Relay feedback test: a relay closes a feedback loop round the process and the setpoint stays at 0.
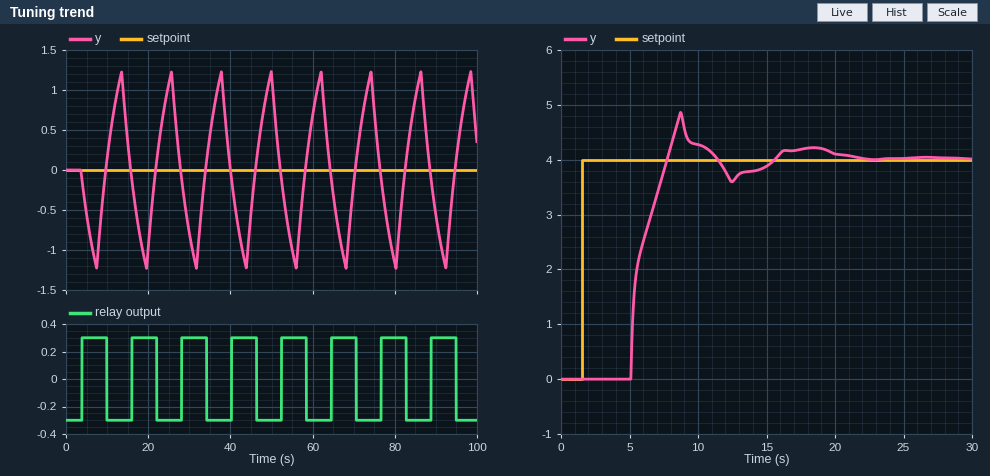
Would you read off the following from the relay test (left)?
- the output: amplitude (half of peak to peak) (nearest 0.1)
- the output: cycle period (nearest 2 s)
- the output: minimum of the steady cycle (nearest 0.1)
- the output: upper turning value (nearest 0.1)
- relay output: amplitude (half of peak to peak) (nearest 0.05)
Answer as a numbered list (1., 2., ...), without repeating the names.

1. 1.2
2. 12 s
3. -1.2
4. 1.2
5. 0.30
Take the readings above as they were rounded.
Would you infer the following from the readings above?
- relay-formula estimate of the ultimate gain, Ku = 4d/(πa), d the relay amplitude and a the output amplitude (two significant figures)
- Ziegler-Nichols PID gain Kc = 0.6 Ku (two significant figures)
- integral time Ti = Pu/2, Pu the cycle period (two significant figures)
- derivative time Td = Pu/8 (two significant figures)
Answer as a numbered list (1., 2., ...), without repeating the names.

1. 0.32
2. 0.19
3. 6.0 s
4. 1.5 s
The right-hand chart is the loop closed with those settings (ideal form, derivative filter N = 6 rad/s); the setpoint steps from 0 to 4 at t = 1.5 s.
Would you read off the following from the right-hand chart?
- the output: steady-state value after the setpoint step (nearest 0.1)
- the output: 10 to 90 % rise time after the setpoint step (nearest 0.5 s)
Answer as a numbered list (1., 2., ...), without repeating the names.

1. 4.0
2. 2.0 s
